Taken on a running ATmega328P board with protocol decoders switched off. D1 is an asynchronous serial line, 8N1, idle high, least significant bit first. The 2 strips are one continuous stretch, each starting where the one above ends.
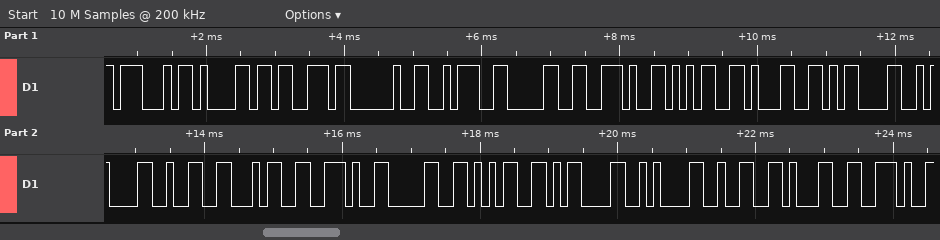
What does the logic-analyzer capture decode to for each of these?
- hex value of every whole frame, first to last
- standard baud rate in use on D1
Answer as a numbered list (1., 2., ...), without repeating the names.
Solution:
1. 47 61 73 20 3A 30 2E 35 31 0D 0A 32 34 2E 30 35 0D 0A 32 31 2E
2. 9600 baud
